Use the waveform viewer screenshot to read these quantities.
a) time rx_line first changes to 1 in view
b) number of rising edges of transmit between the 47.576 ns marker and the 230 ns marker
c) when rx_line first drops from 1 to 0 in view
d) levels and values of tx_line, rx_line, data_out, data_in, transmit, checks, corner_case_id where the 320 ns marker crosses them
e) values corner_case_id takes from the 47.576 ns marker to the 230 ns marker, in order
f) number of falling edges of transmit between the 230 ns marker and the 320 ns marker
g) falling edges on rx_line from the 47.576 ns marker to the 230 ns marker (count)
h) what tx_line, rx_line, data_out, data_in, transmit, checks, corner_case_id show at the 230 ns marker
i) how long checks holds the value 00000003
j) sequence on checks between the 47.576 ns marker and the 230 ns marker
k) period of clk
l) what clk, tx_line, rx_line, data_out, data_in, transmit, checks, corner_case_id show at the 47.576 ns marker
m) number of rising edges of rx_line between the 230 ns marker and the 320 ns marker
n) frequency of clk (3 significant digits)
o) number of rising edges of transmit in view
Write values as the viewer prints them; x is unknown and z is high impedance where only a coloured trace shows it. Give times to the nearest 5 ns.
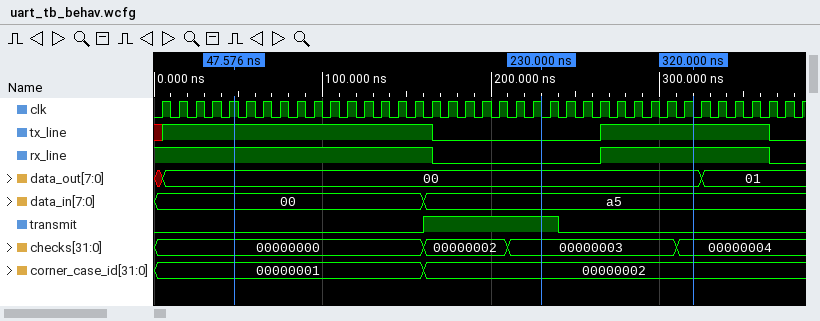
265 ns
1
165 ns
tx_line=1, rx_line=1, data_out=00, data_in=a5, transmit=0, checks=00000004, corner_case_id=00000002
00000001, 00000002
1
1
tx_line=0, rx_line=0, data_out=00, data_in=a5, transmit=1, checks=00000003, corner_case_id=00000002
100 ns
00000000, 00000002, 00000003
10 ns
clk=1, tx_line=1, rx_line=1, data_out=00, data_in=00, transmit=0, checks=00000000, corner_case_id=00000001
1
100 MHz
1
